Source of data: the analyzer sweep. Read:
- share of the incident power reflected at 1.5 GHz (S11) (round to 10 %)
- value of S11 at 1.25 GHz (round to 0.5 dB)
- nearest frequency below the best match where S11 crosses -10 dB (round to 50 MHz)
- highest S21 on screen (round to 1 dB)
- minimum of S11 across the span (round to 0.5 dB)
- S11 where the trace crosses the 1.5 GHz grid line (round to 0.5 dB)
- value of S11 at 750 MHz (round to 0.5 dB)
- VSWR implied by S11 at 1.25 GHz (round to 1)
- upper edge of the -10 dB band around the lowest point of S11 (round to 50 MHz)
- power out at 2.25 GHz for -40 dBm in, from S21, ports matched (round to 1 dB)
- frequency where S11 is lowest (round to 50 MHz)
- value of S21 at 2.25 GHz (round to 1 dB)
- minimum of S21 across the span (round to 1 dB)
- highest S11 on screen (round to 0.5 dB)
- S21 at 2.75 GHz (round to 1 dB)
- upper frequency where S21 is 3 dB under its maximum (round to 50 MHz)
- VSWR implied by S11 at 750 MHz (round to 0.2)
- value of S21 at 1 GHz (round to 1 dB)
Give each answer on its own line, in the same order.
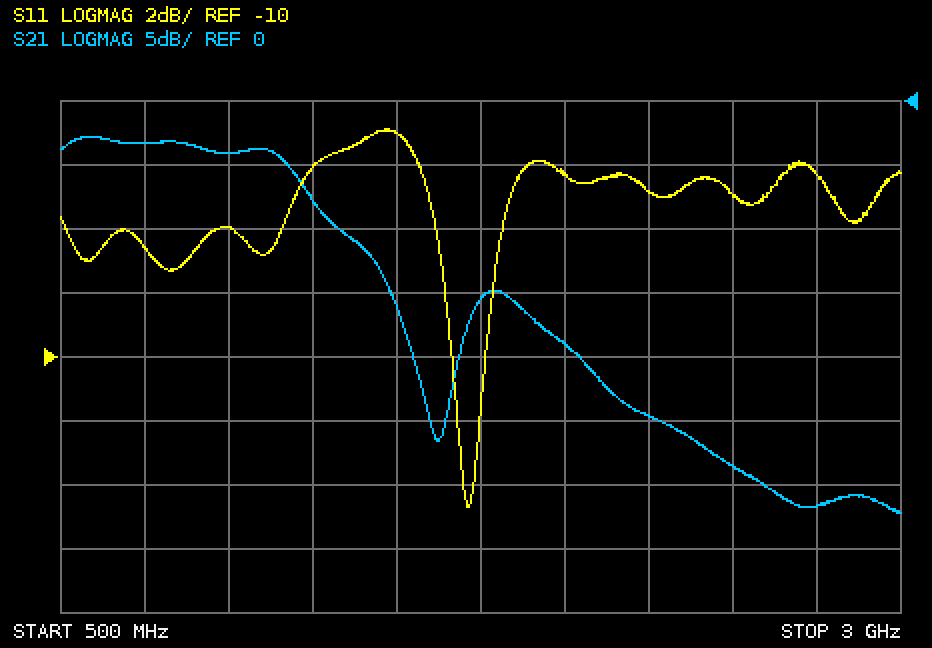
50 %
-4.0 dB
1.65 GHz
-3 dB
-14.5 dB
-3.0 dB
-6.5 dB
4
1.75 GHz
-65 dBm
1.70 GHz
-25 dB
-32 dB
-3.0 dB
-32 dB
1.20 GHz
2.8
-4 dB
